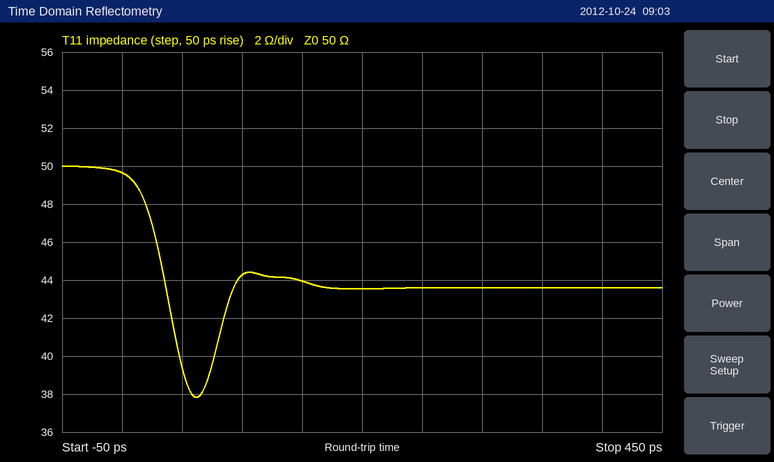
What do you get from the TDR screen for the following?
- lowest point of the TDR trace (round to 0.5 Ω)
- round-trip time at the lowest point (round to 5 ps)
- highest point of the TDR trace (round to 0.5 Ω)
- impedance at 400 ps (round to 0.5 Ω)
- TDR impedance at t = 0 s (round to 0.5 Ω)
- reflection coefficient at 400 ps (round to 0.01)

38.0 Ω
60 ps
50.0 Ω
43.5 Ω
49.5 Ω
-0.07
